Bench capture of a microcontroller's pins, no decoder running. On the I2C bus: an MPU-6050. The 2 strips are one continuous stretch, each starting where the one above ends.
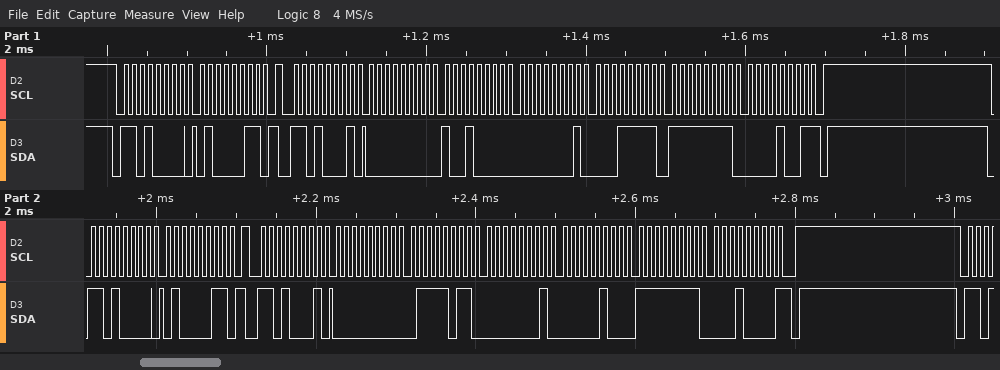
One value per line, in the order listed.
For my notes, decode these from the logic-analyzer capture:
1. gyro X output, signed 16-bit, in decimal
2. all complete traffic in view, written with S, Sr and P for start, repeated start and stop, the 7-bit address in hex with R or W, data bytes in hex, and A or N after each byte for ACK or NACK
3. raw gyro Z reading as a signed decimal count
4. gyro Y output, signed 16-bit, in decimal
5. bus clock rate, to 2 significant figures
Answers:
144
S 68W A 43 A Sr 68R A 00 A 90 A 01 A 1F A FF A 09 N P S 68W A 43 A Sr 68R A 00 A 7B A 01 A 04 A FF A 10 N P
-247
287
100 kHz
